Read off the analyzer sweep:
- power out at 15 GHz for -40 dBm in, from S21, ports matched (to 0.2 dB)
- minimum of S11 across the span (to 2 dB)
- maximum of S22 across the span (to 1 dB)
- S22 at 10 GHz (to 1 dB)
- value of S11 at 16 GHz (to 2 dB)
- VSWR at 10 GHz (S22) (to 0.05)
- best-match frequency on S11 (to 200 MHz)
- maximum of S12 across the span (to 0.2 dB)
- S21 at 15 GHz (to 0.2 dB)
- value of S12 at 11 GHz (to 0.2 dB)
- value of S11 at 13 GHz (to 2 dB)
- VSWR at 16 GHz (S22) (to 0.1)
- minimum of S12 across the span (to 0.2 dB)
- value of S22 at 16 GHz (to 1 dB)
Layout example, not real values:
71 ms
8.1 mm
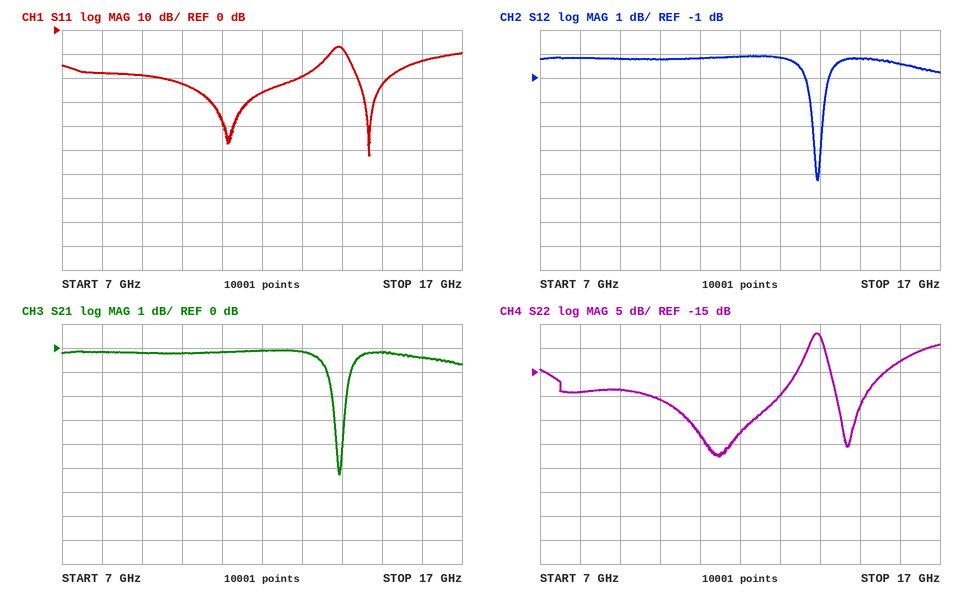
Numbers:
-40.2 dBm
-52 dB
-7 dB
-21 dB
-12 dB
1.20
14.6 GHz
0.0 dB
-0.2 dB
-0.2 dB
-20 dB
1.6
-5.2 dB
-13 dB
